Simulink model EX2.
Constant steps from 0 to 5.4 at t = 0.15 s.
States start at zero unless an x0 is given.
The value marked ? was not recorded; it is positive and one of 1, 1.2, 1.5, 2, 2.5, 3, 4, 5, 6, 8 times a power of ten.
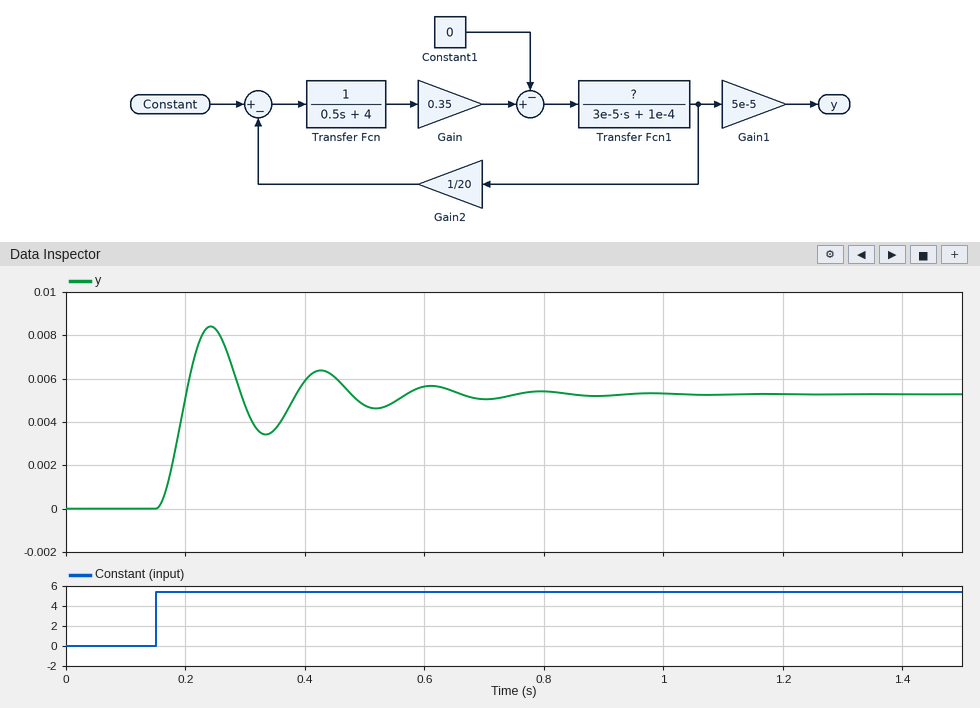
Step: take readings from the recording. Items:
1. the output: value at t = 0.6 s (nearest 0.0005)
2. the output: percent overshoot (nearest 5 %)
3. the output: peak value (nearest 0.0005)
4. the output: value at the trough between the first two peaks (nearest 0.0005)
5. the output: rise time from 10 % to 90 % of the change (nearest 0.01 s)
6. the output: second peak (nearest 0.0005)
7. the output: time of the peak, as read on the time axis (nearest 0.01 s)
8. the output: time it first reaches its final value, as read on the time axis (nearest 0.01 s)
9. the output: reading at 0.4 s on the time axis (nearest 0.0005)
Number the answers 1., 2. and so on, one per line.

1. 0.0055
2. 60 %
3. 0.0085
4. 0.0035
5. 0.03 s
6. 0.0065
7. 0.24 s
8. 0.20 s
9. 0.0060
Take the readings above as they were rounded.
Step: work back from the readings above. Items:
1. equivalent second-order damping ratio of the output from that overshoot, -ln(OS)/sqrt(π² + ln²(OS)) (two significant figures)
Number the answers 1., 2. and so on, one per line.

1. 0.16
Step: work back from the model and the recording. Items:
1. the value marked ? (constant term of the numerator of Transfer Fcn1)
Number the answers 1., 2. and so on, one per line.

1. 1
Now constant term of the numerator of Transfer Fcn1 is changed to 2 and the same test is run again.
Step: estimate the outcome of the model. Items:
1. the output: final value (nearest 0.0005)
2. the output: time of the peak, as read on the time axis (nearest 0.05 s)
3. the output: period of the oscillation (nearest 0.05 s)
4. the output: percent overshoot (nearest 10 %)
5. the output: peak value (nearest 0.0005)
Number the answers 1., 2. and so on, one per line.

1. 0.0055
2. 0.20 s
3. 0.15 s
4. 70 %
5. 0.0090
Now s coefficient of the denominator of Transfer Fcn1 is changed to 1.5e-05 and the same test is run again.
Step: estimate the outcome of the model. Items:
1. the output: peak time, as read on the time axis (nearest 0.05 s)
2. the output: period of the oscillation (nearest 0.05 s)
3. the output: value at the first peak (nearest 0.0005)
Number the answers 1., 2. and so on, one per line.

1. 0.20 s
2. 0.15 s
3. 0.0085
